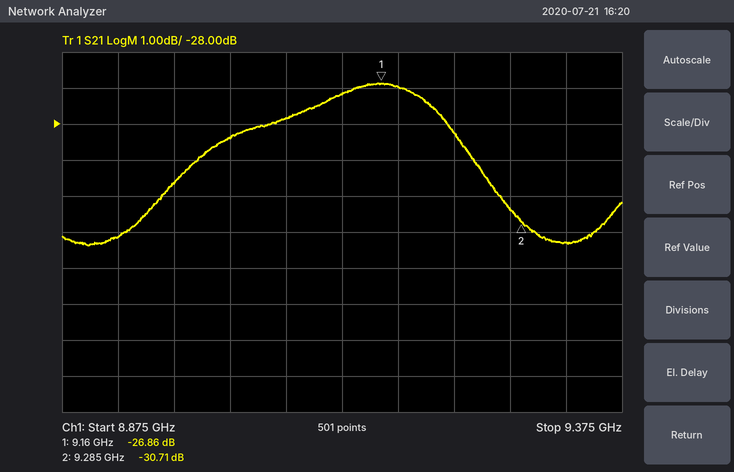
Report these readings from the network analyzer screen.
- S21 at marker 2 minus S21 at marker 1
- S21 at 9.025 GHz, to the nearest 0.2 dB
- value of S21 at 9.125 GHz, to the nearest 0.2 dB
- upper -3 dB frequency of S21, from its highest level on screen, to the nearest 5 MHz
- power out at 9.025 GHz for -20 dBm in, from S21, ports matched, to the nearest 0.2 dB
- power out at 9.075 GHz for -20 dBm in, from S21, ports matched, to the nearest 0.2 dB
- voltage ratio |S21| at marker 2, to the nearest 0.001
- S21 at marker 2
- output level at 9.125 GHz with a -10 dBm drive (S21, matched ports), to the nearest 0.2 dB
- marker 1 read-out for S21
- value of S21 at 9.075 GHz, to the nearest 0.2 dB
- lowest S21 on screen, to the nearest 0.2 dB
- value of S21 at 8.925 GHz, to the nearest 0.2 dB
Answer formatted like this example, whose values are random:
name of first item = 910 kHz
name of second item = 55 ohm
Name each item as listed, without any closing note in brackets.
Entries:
S21 at marker 2 minus S21 at marker 1 = -3.85 dB
S21 at 9.025 GHz, to the nearest 0.2 dB = -28.4 dB
value of S21 at 9.125 GHz, to the nearest 0.2 dB = -27.2 dB
upper -3 dB frequency of S21, from its highest level on screen, to the nearest 5 MHz = 9.260 GHz
power out at 9.025 GHz for -20 dBm in, from S21, ports matched, to the nearest 0.2 dB = -48.4 dBm
power out at 9.075 GHz for -20 dBm in, from S21, ports matched, to the nearest 0.2 dB = -47.8 dBm
voltage ratio |S21| at marker 2, to the nearest 0.001 = 0.029
S21 at marker 2 = -30.71 dB
output level at 9.125 GHz with a -10 dBm drive (S21, matched ports), to the nearest 0.2 dB = -37.2 dBm
marker 1 read-out for S21 = -26.86 dB
value of S21 at 9.075 GHz, to the nearest 0.2 dB = -27.8 dB
lowest S21 on screen, to the nearest 0.2 dB = -31.4 dB
value of S21 at 8.925 GHz, to the nearest 0.2 dB = -31.2 dB
